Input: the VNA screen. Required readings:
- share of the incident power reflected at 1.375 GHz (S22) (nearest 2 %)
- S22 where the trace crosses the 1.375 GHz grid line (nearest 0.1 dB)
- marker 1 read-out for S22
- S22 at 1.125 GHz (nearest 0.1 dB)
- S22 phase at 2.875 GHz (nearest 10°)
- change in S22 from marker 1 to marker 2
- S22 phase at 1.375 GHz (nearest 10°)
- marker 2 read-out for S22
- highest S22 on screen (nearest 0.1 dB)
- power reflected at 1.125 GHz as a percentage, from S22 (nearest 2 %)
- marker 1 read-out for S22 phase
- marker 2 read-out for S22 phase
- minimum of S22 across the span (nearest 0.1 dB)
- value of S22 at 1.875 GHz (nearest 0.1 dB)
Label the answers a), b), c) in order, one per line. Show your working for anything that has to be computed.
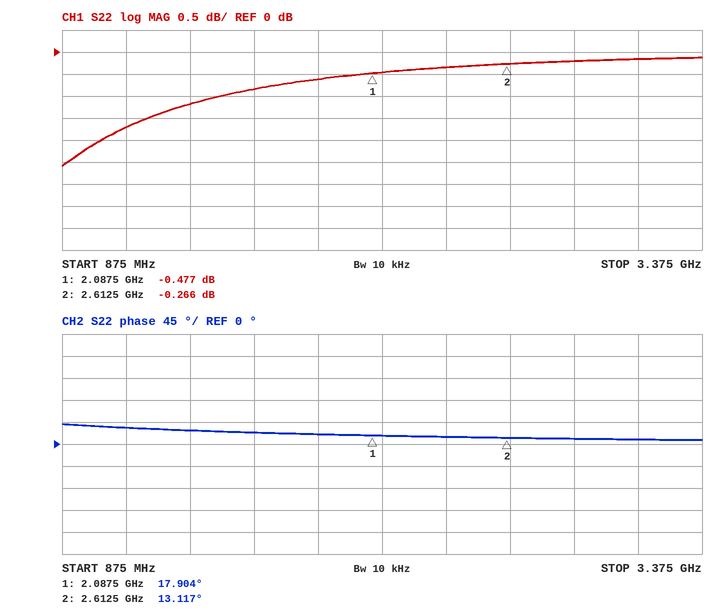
a) 10^(-1.2/10) ≈ 76 %
b) -1.2 dB
c) -0.477 dB
d) -1.7 dB
e) 10°
f) -0.266 − (-0.477) = 0.211 dB
g) 30°
h) -0.266 dB
i) -0.1 dB
j) 10^(-1.7/10) ≈ 68 %
k) 17.904°
l) 13.117°
m) -2.6 dB
n) -0.6 dB
